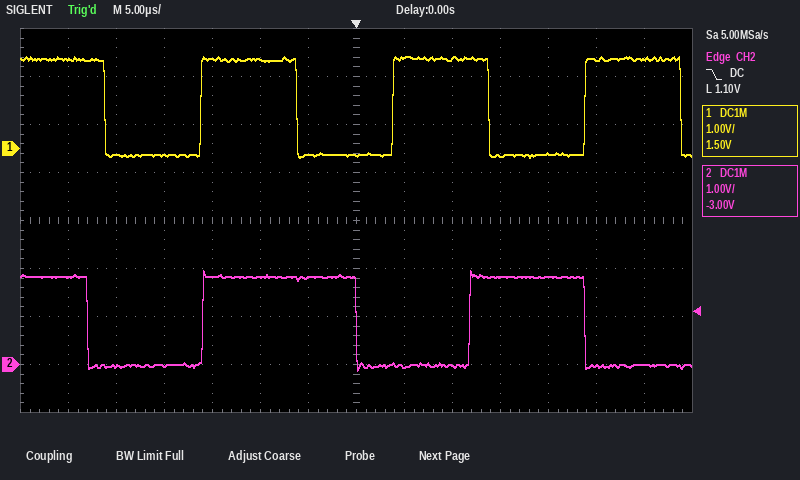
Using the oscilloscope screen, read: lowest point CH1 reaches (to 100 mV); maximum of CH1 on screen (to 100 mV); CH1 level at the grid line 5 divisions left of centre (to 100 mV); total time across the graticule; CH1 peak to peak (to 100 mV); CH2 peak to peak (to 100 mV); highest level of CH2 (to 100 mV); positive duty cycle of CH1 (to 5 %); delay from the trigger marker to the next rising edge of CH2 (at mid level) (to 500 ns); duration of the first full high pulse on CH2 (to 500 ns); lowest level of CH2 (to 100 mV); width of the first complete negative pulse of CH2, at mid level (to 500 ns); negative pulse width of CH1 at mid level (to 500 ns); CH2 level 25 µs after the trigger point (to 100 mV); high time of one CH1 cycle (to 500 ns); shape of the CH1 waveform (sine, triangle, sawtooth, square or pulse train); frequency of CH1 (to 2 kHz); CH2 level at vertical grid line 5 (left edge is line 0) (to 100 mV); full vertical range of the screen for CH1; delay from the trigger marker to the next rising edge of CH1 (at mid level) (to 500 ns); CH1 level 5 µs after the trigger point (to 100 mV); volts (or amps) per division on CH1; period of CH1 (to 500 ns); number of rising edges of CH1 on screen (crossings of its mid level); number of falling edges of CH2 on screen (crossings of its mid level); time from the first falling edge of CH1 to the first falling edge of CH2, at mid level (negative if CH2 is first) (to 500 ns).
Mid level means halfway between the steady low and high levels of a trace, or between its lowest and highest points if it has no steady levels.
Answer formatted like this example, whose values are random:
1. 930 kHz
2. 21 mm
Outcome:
1. -200 mV
2. 1.9 V
3. -100 mV
4. 70 µs
5. 2.1 V
6. 2.1 V
7. 2.0 V
8. 50 %
9. 12.0 µs
10. 16.0 µs
11. -100 mV
12. 12.0 µs
13. 10.0 µs
14. 0.0 V
15. 10.0 µs
16. square
17. 50 kHz
18. 1.8 V
19. 8 V
20. 4.0 µs
21. 1.9 V
22. 1 V
23. 20.0 µs
24. 3
25. 3
26. -2.0 µs
